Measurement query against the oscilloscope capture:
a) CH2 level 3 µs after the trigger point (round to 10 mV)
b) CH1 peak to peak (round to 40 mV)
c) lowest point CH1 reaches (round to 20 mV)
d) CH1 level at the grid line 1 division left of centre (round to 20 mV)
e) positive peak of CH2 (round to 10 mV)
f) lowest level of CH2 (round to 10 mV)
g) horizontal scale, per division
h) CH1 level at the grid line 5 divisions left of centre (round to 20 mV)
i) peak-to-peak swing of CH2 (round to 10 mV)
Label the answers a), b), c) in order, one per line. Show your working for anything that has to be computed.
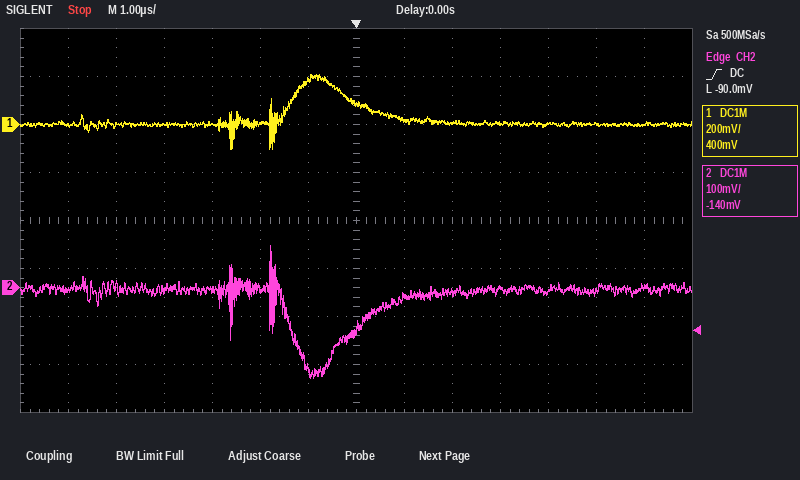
a) 0 mV
b) 320 mV
c) -100 mV
d) 180 mV
e) 90 mV
f) -190 mV
g) 1 µs
h) 0 mV
i) 90 mV − (-190 mV) = 280 mV
